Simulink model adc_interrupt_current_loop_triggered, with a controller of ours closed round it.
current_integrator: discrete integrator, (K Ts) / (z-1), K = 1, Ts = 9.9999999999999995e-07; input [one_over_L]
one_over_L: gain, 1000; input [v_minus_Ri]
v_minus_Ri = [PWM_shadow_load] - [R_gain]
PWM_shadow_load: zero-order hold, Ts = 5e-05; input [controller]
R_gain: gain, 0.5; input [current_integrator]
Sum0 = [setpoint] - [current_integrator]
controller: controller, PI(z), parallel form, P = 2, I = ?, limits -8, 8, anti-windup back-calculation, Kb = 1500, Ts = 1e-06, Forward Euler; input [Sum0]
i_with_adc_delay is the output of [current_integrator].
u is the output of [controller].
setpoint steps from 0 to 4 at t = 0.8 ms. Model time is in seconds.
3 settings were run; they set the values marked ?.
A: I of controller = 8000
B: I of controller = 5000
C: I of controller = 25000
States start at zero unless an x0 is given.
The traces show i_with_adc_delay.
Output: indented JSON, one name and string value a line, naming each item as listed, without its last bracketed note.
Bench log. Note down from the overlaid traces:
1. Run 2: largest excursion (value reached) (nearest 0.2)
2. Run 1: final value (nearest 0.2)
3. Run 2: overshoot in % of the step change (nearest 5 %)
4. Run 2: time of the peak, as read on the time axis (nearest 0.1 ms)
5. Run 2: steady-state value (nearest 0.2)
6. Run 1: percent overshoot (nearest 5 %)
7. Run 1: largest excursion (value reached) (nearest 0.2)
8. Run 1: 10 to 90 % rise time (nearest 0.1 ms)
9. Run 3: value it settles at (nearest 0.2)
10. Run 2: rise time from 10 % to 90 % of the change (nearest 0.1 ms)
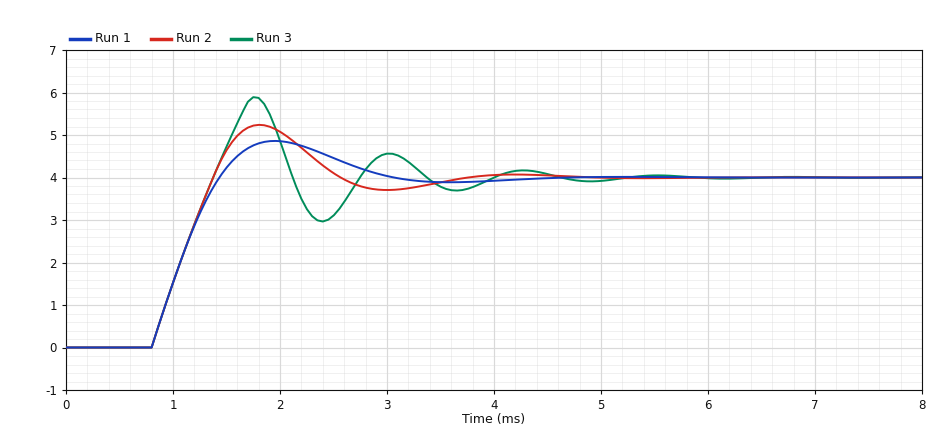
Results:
{
  "Run 2: largest excursion (value reached)": "5.2",
  "Run 1: final value": "4.0",
  "Run 2: overshoot in % of the step change": "30 %",
  "Run 2: time of the peak, as read on the time axis": "1.8 ms",
  "Run 2: steady-state value": "4.0",
  "Run 1: percent overshoot": "20 %",
  "Run 1: largest excursion (value reached)": "4.8",
  "Run 1: 10 to 90 % rise time": "0.5 ms",
  "Run 3: value it settles at": "4.0",
  "Run 2: rise time from 10 % to 90 % of the change": "0.5 ms"
}
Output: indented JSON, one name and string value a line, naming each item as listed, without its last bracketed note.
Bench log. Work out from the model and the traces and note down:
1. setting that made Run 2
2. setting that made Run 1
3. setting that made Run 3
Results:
{
  "setting that made Run 2": "A",
  "setting that made Run 1": "B",
  "setting that made Run 3": "C"
}
